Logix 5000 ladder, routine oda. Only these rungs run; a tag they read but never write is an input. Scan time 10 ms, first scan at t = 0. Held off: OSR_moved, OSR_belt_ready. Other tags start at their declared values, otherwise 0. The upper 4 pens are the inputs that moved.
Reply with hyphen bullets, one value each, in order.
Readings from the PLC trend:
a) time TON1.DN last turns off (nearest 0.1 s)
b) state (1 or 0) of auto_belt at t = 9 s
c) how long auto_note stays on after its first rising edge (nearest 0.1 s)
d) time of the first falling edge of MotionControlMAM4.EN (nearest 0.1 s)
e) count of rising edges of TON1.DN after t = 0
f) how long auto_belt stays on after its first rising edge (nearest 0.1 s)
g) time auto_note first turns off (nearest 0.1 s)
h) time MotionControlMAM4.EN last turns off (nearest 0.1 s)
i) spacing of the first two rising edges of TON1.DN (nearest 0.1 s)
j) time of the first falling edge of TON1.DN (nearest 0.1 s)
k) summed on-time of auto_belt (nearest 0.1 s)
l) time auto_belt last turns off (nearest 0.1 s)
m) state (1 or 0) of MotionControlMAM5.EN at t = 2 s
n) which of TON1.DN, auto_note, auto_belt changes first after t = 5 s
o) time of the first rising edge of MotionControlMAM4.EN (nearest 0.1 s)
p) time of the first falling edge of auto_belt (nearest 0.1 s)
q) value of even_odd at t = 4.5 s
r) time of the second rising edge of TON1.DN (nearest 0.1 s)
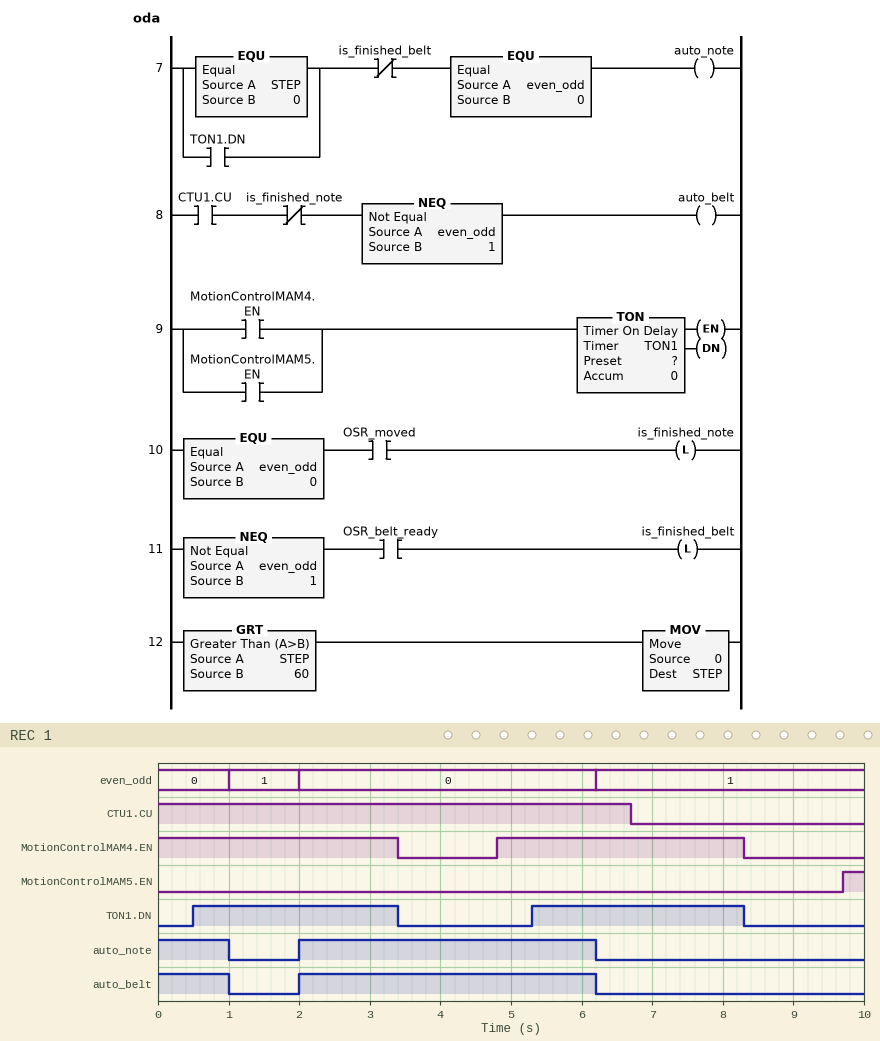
- 8.3 s
- 0
- 4.2 s
- 3.4 s
- 2
- 4.2 s
- 1.0 s
- 8.3 s
- 4.8 s
- 3.4 s
- 5.2 s
- 6.2 s
- 0
- TON1.DN
- 4.8 s
- 1.0 s
- 0
- 5.3 s
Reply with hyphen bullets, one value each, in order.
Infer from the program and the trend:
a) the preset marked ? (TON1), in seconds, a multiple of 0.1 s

- 0.5 s
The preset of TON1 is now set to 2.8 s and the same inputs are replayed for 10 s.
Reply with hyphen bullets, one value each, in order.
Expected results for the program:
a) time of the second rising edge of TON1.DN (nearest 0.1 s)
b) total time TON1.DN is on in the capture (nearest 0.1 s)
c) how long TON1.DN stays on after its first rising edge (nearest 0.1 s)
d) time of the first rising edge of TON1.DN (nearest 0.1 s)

- 7.6 s
- 1.3 s
- 0.6 s
- 2.8 s
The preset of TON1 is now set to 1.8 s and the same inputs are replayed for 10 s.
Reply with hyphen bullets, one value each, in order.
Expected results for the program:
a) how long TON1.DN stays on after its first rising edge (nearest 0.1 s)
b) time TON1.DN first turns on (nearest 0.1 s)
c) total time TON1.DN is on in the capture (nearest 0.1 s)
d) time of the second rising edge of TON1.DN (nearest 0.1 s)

- 1.6 s
- 1.8 s
- 3.3 s
- 6.6 s
